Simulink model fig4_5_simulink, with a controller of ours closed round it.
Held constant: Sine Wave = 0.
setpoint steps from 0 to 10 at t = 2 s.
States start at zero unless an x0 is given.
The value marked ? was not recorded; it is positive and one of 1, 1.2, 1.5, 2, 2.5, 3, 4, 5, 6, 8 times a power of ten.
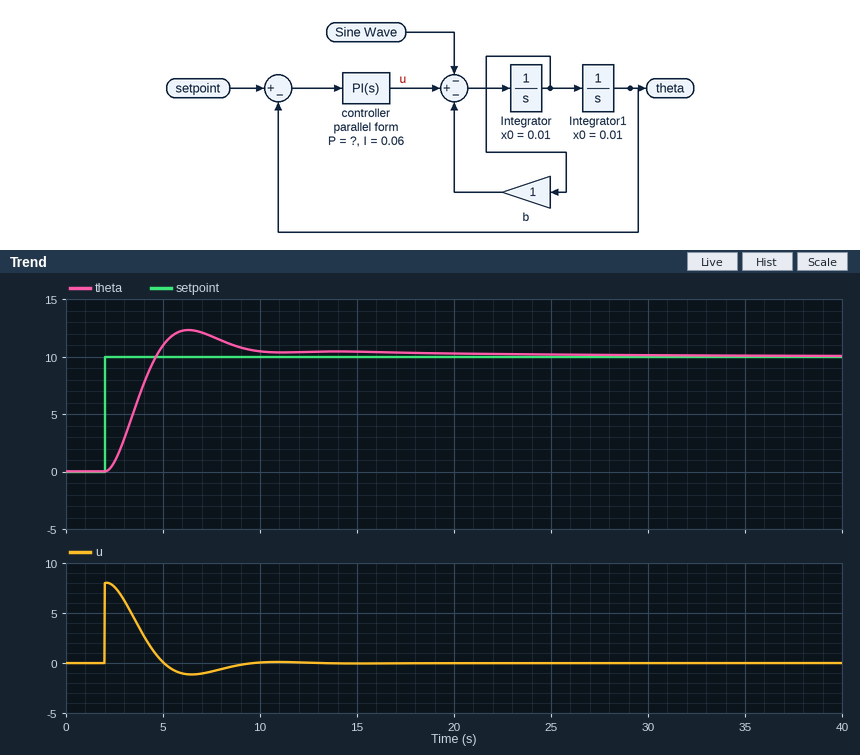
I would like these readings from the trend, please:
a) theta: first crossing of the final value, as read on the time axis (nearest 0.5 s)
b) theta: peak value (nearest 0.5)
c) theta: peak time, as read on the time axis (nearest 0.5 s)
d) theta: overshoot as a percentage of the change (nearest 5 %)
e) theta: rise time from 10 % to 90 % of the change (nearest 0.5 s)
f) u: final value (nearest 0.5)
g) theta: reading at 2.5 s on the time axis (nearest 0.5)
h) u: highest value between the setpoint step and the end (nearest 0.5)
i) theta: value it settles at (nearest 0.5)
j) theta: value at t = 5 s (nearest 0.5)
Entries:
4.5 s
12.5
6.5 s
25 %
2.0 s
0.0
1.0
8.0
10.0
11.0
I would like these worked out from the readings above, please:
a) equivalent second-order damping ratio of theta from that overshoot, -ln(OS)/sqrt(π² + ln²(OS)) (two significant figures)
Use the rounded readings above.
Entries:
0.40
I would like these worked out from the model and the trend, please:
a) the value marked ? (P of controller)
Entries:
0.8
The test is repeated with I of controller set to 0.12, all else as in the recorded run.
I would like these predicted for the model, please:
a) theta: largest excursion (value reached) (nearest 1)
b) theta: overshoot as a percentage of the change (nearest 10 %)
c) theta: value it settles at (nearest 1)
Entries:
13
30 %
10
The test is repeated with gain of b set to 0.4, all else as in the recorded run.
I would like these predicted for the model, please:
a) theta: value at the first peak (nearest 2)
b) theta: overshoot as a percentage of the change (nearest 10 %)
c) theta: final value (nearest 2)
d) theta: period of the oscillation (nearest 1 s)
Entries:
16
60 %
10
7 s
